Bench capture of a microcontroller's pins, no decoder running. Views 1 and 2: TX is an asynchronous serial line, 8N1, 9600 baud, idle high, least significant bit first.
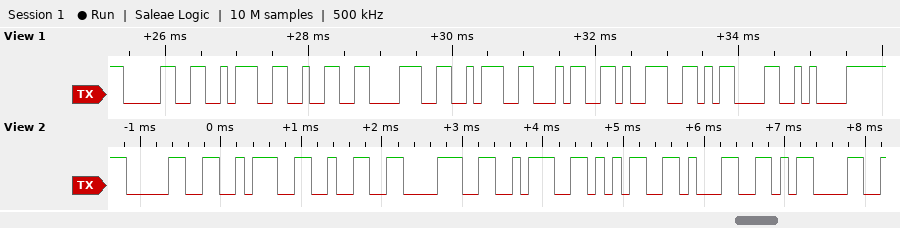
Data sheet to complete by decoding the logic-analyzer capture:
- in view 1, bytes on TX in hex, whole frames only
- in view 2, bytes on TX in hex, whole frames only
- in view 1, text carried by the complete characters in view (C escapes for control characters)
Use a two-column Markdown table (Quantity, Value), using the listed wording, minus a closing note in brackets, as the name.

| Quantity | Value |
|---|---|
| in view 1, bytes on TX in hex, whole frames only | 0x30 0x3A 0x32 0x38 0x3A 0x34 0x39 0x0D 0x0A |
| in view 2, bytes on TX in hex, whole frames only | 0x30 0x3A 0x32 0x38 0x3A 0x35 0x31 0x0D |
| in view 1, text carried by the complete characters in view | "0:28:49\r\n" |
